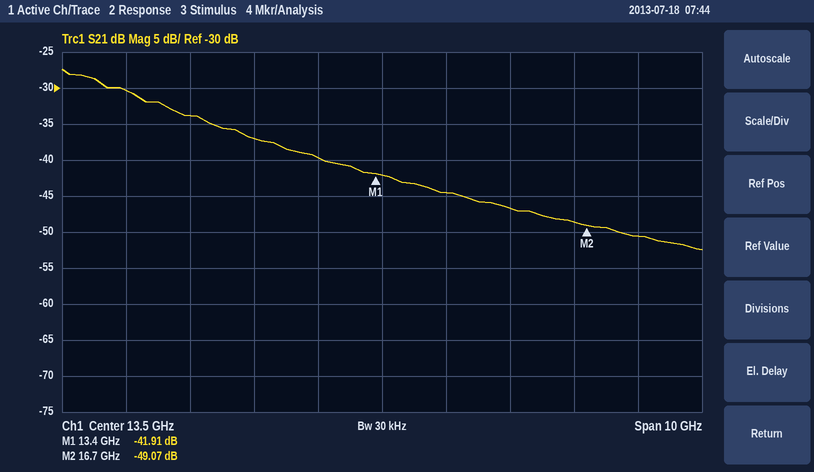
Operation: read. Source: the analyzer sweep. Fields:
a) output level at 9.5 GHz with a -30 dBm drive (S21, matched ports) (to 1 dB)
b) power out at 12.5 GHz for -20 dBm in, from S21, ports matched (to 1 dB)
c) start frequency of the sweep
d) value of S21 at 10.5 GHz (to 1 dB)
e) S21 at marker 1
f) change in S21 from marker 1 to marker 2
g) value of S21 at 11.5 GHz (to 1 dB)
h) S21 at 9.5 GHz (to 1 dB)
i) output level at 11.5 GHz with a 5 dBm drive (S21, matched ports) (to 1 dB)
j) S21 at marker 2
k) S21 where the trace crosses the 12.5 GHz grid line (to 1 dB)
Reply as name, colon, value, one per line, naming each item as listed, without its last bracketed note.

output level at 9.5 GHz with a -30 dBm drive (S21, matched ports): -60 dBm
power out at 12.5 GHz for -20 dBm in, from S21, ports matched: -60 dBm
start frequency of the sweep: 8.5 GHz
value of S21 at 10.5 GHz: -34 dB
S21 at marker 1: -41.91 dB
change in S21 from marker 1 to marker 2: -7.16 dB
value of S21 at 11.5 GHz: -37 dB
S21 at 9.5 GHz: -30 dB
output level at 11.5 GHz with a 5 dBm drive (S21, matched ports): -32 dBm
S21 at marker 2: -49.07 dB
S21 where the trace crosses the 12.5 GHz grid line: -40 dB
